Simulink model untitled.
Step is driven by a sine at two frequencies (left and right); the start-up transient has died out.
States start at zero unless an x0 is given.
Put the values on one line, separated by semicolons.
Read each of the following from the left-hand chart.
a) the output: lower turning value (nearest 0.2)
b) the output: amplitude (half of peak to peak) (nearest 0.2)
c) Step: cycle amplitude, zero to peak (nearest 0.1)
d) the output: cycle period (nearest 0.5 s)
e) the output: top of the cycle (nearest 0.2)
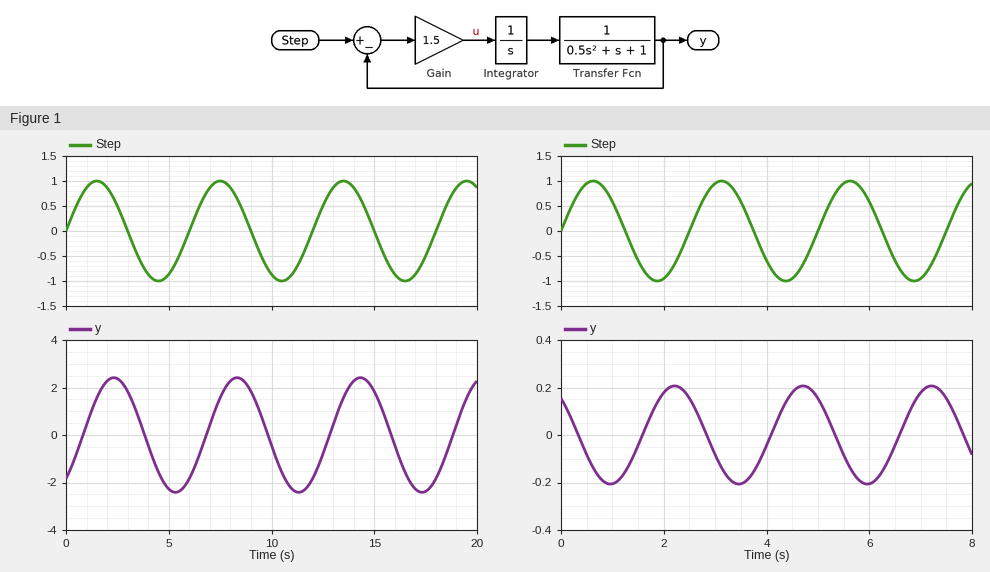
-2.4; 2.4; 1.0; 6.0 s; 2.4
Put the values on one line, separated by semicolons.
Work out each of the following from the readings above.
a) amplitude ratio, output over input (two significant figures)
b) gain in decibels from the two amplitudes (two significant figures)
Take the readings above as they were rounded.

2.4; 7.6 dB
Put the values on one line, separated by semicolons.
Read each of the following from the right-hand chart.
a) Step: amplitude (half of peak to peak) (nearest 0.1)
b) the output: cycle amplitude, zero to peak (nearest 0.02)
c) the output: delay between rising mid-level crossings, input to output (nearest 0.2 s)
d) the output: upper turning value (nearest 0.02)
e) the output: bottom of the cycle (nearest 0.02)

1.0; 0.20; 1.6 s; 0.20; -0.20
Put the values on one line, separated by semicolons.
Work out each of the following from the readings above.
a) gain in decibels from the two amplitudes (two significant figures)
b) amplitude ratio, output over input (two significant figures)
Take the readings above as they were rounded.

-14 dB; 0.20
